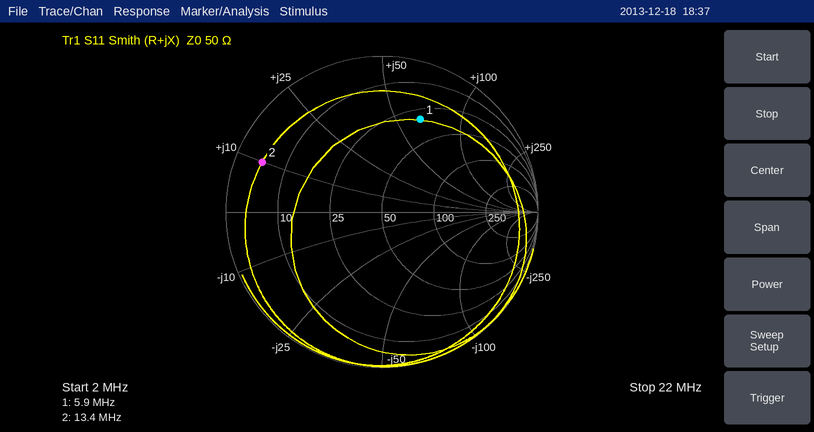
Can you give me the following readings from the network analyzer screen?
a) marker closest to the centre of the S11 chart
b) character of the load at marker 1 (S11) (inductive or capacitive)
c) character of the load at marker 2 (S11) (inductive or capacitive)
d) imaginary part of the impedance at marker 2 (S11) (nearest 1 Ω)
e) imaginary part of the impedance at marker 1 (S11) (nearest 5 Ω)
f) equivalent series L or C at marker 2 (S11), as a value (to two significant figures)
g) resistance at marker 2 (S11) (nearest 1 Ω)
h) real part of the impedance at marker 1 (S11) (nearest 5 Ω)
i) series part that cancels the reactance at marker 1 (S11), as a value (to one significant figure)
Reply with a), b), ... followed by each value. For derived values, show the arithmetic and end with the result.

a) marker 1
b) inductive
c) inductive
d) +10 Ω
e) +65 Ω
f) L = 10 Ω/(2π × 13.4 MHz) ≈ 119 nH, so 120 nH to two significant figures
g) 5 Ω
h) 30 Ω
i) C = 1/(2π × 5.9 MHz × 65 Ω) ≈ 415 pF, so 400 pF to one significant figure
